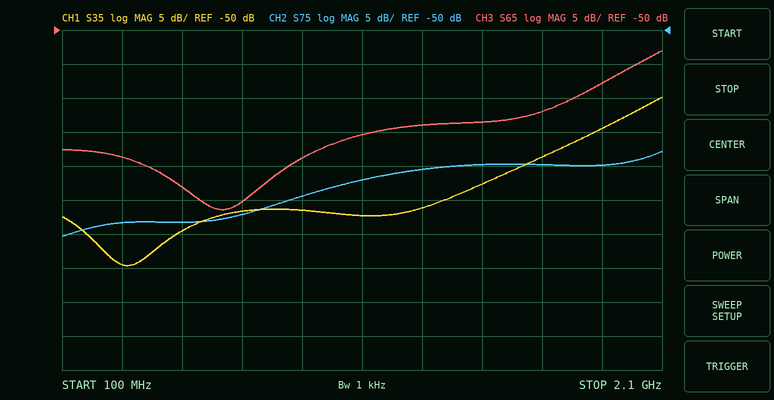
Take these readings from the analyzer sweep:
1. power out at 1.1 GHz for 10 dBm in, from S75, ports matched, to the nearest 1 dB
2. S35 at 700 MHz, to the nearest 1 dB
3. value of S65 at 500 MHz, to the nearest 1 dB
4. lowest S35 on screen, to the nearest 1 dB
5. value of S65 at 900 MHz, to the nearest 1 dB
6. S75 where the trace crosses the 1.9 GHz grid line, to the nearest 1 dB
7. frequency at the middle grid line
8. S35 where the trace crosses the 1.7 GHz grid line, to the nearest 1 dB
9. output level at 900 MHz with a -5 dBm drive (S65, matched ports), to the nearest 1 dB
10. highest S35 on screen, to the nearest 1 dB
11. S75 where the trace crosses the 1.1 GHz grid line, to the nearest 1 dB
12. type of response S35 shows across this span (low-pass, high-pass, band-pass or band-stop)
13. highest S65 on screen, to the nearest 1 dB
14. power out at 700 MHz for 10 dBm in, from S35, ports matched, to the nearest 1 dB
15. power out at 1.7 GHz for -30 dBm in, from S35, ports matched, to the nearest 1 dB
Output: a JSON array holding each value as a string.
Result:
["-62 dBm", "-77 dB", "-73 dB", "-85 dB", "-69 dB", "-70 dB", "1.1 GHz", "-69 dB", "-74 dBm", "-60 dB", "-72 dB", "high-pass", "-53 dB", "-67 dBm", "-99 dBm"]
